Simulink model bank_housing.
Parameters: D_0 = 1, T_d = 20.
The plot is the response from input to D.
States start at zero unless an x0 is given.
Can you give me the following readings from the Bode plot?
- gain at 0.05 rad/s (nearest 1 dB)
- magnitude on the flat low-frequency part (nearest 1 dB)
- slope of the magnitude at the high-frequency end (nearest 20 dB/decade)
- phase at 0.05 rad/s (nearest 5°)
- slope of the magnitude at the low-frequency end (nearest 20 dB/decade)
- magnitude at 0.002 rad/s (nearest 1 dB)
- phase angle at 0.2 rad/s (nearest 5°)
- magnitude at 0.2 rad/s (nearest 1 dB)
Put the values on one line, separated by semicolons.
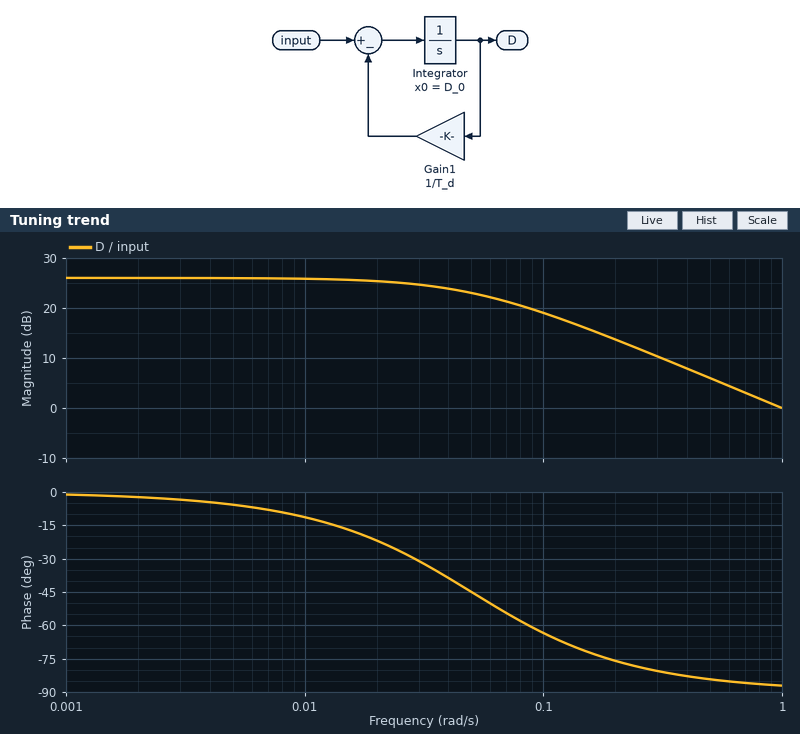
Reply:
23 dB; 26 dB; -20 dB/decade; -45°; 0 dB/decade; 26 dB; -75°; 14 dB
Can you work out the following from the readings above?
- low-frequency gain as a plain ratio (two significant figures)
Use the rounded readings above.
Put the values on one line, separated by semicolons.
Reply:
20
